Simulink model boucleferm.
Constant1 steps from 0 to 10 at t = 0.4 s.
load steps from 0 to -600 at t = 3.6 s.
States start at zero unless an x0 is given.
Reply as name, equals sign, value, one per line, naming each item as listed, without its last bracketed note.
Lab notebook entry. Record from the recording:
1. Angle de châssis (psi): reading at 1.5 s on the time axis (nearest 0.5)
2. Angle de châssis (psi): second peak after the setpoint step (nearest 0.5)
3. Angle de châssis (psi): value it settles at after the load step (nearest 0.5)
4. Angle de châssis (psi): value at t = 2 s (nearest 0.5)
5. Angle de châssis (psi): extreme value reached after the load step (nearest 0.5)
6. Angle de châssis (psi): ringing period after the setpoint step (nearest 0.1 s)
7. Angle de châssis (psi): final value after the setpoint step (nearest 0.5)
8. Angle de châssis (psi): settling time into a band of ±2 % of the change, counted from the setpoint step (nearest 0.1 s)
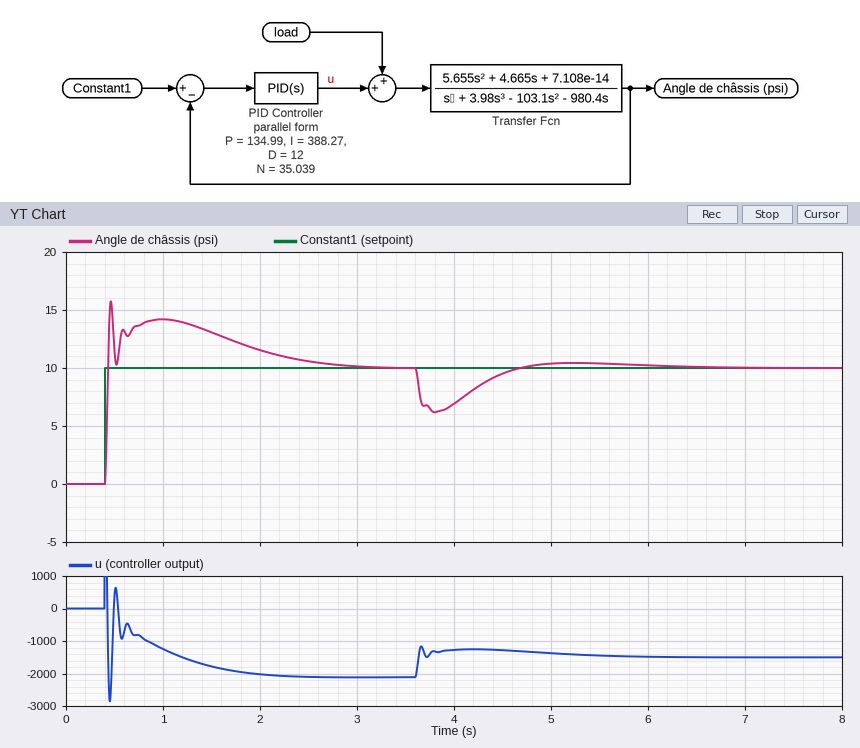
Angle de châssis (psi): reading at 1.5 s on the time axis = 13.0
Angle de châssis (psi): second peak after the setpoint step = 14.0
Angle de châssis (psi): value it settles at after the load step = 10.0
Angle de châssis (psi): value at t = 2 s = 11.5
Angle de châssis (psi): extreme value reached after the load step = 6.0
Angle de châssis (psi): ringing period after the setpoint step = 0.5 s
Angle de châssis (psi): final value after the setpoint step = 10.0
Angle de châssis (psi): settling time into a band of ±2 % of the change, counted from the setpoint step = 2.5 s
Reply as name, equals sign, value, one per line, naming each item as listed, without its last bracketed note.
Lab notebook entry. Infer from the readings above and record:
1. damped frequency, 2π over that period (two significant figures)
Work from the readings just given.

damped frequency, 2π over that period = 13 rad/s
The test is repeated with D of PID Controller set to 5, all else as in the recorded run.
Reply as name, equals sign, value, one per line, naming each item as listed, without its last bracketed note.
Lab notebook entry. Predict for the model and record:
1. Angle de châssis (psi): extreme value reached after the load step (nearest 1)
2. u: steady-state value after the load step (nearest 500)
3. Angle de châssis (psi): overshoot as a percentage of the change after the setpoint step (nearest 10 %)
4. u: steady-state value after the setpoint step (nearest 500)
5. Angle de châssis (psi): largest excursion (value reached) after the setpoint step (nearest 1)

Angle de châssis (psi): extreme value reached after the load step = 5
u: steady-state value after the load step = -1500
Angle de châssis (psi): overshoot as a percentage of the change after the setpoint step = 80 %
u: steady-state value after the setpoint step = -2000
Angle de châssis (psi): largest excursion (value reached) after the setpoint step = 18
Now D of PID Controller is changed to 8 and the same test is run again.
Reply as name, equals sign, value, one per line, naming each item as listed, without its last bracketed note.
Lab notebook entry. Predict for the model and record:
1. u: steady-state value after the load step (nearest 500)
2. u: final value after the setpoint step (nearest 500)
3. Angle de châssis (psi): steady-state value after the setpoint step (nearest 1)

u: steady-state value after the load step = -1500
u: final value after the setpoint step = -2000
Angle de châssis (psi): steady-state value after the setpoint step = 10
